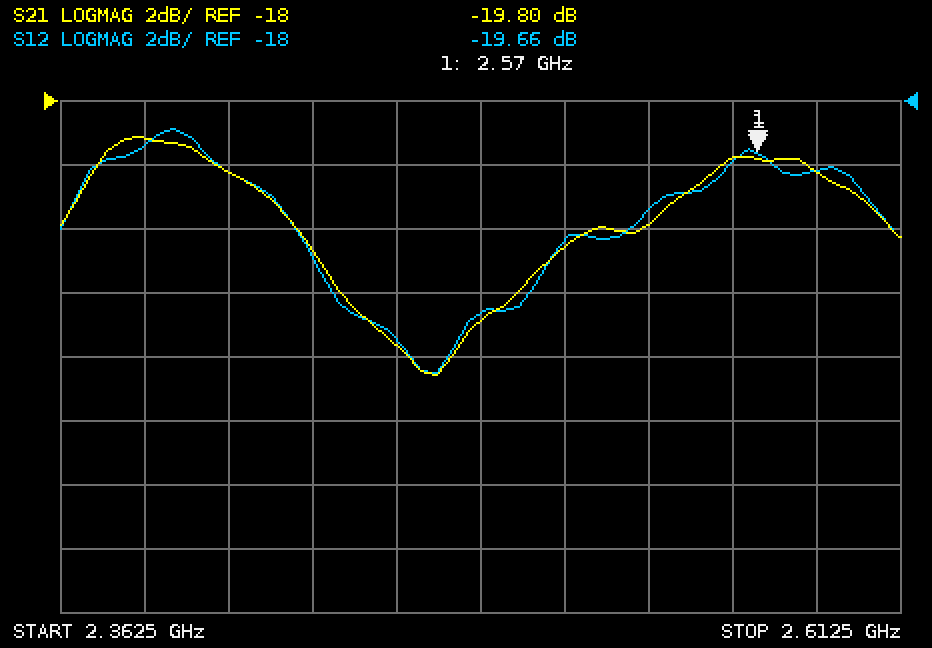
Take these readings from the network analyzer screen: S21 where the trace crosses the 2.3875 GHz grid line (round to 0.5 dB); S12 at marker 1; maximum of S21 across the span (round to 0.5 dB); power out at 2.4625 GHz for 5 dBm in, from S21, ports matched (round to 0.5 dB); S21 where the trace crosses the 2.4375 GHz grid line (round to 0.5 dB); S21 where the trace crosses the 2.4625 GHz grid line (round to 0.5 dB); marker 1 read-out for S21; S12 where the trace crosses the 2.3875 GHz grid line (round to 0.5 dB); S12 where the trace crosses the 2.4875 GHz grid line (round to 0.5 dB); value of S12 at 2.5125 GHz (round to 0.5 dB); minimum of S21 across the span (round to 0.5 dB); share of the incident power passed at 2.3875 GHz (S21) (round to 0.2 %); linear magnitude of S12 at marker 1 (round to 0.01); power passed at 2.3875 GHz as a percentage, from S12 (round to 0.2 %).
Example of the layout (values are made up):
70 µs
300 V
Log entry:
-19.0 dB
-19.66 dB
-19.0 dB
-20.5 dBm
-22.5 dB
-25.5 dB
-19.80 dB
-19.5 dB
-24.5 dB
-22.5 dB
-26.5 dB
1.2 %
0.10
1.2 %
